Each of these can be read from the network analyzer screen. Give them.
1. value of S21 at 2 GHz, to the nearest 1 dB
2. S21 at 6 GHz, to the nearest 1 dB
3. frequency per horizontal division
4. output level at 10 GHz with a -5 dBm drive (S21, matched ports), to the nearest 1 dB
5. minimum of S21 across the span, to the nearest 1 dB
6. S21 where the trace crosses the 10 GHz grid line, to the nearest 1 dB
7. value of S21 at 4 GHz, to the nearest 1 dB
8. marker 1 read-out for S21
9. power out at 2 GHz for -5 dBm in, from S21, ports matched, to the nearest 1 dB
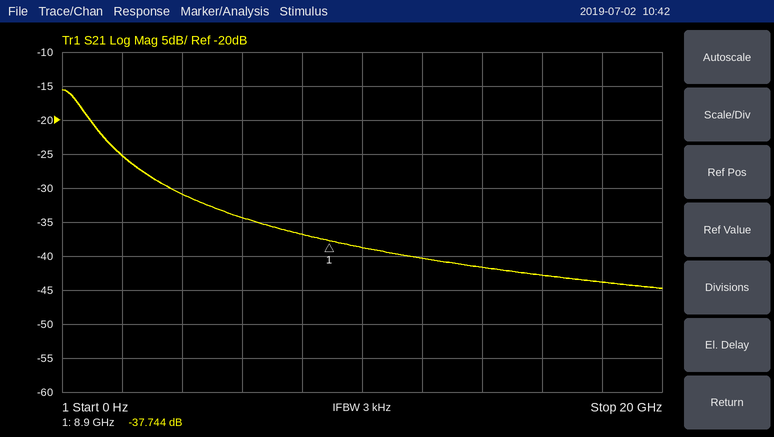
-25 dB
-34 dB
2 GHz
-44 dBm
-45 dB
-39 dB
-31 dB
-37.744 dB
-30 dBm
